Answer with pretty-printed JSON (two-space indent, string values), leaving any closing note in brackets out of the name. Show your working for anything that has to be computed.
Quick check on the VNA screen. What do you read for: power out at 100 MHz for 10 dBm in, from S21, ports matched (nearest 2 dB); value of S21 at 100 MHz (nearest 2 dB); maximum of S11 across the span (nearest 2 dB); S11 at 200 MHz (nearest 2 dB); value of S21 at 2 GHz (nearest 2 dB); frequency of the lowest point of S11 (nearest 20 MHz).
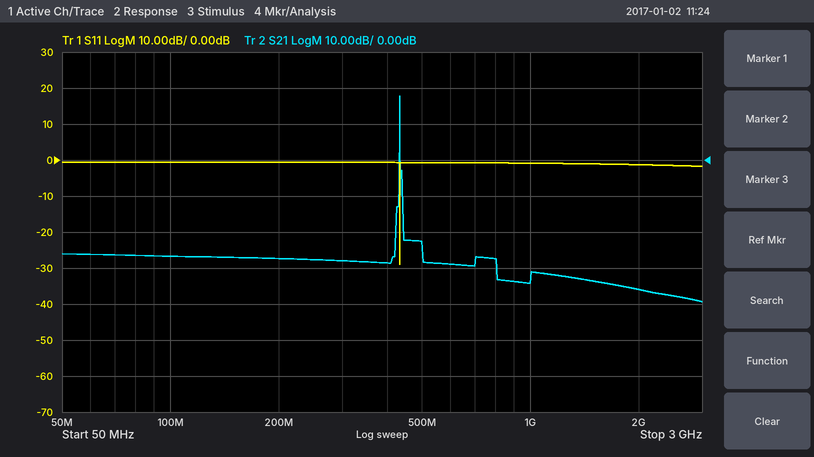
{
  "power out at 100 MHz for 10 dBm in, from S21, ports matched": "10 dBm + (-26 dB) = -16 dBm",
  "value of S21 at 100 MHz": "-26 dB",
  "maximum of S11 across the span": "0 dB",
  "S11 at 200 MHz": "0 dB",
  "value of S21 at 2 GHz": "-36 dB",
  "frequency of the lowest point of S11": "440 MHz"
}
